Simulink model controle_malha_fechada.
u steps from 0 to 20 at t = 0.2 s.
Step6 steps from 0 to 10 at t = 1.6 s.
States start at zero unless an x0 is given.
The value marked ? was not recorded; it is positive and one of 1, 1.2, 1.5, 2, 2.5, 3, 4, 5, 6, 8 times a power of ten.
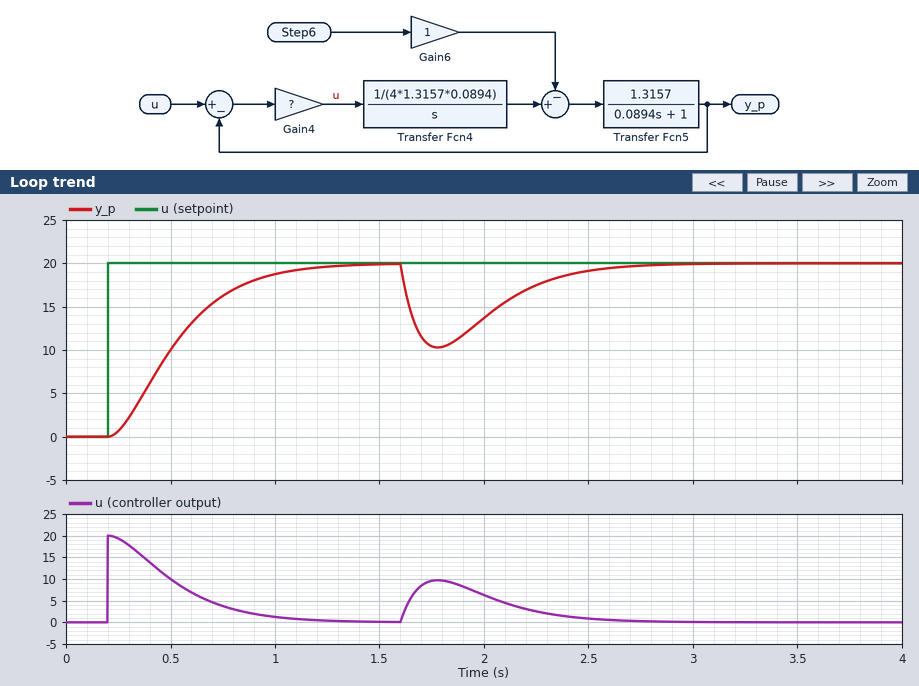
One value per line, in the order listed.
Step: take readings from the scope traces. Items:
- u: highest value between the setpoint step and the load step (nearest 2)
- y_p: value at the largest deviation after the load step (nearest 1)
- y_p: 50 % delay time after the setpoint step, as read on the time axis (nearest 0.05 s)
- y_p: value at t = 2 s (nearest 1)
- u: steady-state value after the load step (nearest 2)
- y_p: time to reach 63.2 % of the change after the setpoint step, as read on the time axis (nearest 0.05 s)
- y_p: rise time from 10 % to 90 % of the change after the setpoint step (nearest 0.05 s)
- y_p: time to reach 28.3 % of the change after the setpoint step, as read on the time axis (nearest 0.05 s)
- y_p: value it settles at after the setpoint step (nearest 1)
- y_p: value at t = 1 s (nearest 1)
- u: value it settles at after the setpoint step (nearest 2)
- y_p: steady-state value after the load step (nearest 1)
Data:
20
10
0.50 s
14
0
0.60 s
0.60 s
0.40 s
20
19
0
20
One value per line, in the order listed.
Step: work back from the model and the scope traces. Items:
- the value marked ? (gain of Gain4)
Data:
1
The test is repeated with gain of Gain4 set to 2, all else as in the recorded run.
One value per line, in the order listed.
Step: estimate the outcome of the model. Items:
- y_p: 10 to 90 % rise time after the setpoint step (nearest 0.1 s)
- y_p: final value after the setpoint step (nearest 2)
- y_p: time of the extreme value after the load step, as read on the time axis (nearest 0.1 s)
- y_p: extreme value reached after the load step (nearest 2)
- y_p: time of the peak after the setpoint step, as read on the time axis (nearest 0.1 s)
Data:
0.3 s
20
1.7 s
12
0.8 s
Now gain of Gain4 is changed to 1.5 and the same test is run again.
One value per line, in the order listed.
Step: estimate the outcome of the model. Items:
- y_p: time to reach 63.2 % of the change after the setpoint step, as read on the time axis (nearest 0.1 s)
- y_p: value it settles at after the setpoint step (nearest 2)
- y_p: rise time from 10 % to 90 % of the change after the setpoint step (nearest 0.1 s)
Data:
0.5 s
20
0.4 s
